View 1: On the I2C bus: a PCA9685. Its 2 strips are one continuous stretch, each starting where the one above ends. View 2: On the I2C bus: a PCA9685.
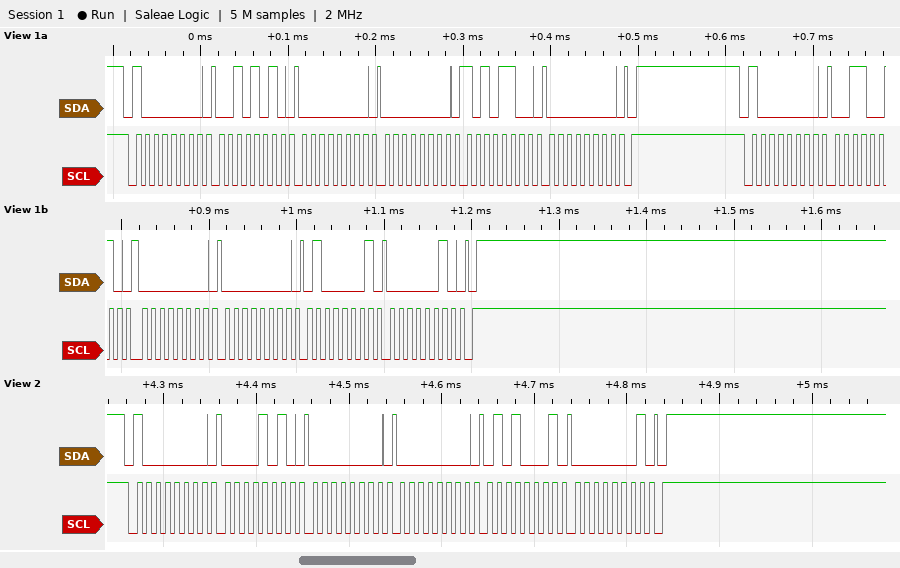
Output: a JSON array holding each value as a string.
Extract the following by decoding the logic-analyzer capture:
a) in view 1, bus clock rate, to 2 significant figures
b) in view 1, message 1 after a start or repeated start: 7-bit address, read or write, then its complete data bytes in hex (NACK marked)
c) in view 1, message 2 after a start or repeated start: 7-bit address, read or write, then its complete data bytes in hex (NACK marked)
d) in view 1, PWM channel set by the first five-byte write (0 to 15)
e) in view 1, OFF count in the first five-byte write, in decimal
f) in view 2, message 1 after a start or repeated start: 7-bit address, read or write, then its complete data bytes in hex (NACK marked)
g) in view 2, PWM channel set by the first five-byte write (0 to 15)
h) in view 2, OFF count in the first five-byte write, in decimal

["100 kHz", "0x40 write: 2A 00 00 AC 00", "0x40 write: 32 00 00 41 02", "9", "172", "0x40 write: 0A 00 00 51 01", "1", "337"]
